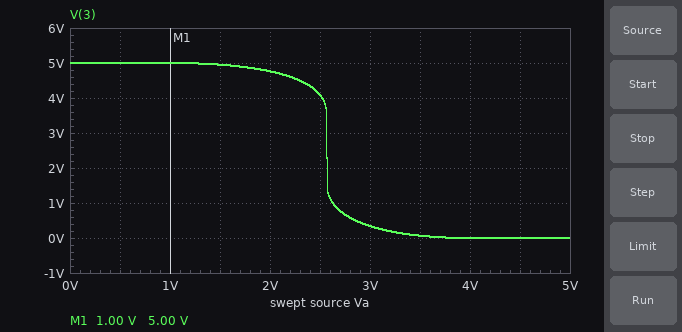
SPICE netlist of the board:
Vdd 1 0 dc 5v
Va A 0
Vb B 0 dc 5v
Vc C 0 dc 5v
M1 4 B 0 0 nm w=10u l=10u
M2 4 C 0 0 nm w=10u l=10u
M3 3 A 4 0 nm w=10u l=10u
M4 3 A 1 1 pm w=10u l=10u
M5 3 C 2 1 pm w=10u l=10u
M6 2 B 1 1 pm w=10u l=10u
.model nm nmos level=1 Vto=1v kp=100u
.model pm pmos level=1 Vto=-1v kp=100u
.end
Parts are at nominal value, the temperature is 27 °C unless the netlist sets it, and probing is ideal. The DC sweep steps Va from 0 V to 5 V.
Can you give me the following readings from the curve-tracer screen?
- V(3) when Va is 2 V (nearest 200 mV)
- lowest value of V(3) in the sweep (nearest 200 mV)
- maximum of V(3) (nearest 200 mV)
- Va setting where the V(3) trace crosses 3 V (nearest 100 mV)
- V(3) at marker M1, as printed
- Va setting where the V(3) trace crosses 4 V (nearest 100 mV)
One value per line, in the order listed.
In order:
4.8 V
0 V
5.0 V
2.6 V
5.00 V
2.5 V
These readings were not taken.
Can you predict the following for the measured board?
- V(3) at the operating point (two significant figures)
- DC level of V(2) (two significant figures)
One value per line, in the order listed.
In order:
5.0 V
5.0 V
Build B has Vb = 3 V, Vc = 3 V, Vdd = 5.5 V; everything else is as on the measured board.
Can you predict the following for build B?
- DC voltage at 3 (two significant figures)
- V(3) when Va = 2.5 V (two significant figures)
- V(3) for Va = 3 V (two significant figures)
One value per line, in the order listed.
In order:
5.5 V
5.2 V
4.7 V
